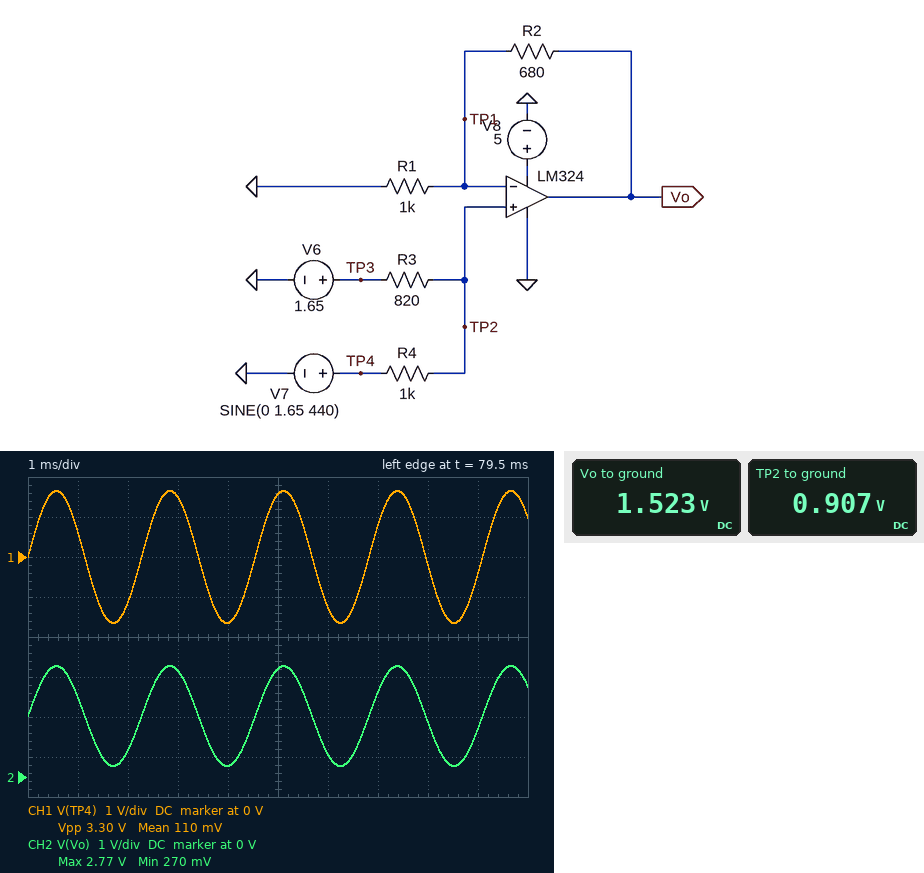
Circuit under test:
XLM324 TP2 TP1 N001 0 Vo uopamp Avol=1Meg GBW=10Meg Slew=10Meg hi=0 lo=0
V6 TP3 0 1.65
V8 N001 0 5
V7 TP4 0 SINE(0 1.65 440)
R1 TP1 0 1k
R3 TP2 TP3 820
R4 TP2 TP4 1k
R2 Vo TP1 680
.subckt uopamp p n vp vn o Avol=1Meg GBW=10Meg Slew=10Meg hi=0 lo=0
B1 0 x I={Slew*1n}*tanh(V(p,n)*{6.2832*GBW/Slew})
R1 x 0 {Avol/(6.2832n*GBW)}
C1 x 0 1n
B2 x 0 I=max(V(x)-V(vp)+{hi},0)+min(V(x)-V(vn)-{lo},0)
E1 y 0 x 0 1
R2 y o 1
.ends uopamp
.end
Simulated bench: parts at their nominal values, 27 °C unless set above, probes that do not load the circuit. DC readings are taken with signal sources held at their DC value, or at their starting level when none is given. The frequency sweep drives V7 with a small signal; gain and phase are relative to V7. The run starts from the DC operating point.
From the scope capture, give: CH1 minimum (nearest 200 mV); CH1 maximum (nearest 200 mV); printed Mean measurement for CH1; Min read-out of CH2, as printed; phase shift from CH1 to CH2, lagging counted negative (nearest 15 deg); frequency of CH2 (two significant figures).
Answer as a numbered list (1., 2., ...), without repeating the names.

1. -1.6 V
2. 1.6 V
3. 110 mV
4. 270 mV
5. 0 deg
6. 440 Hz
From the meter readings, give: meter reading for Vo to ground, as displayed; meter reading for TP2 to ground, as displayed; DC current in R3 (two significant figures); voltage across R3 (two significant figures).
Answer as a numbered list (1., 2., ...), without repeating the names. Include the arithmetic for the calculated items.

1. 1.523 V
2. 0.907 V
3. (1.65 V - 907 mV) / 820 Ω = 910 µA
4. 1.65 V - 907 mV = 740 mV
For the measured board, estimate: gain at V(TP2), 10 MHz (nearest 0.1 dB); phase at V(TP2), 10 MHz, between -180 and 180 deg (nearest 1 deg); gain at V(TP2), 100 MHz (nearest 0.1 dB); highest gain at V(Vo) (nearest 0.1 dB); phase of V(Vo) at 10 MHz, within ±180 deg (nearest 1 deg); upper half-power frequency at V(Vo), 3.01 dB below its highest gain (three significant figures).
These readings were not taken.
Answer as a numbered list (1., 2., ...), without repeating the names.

1. -6.9 dB
2. 0 deg
3. -6.9 dB
4. -2.4 dB
5. -59 deg
6. 5.95 MHz
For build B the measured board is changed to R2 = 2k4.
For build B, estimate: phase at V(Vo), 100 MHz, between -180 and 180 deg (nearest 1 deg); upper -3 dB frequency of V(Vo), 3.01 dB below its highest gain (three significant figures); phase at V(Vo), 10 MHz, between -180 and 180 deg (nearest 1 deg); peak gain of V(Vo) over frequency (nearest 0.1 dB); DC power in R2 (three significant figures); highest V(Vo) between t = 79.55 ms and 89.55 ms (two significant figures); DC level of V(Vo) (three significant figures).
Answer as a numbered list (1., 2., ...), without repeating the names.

1. -88 deg
2. 2.94 MHz
3. -74 deg
4. 3.7 dB
5. 1.97 mW
6. 5.0 V
7. 3.08 V
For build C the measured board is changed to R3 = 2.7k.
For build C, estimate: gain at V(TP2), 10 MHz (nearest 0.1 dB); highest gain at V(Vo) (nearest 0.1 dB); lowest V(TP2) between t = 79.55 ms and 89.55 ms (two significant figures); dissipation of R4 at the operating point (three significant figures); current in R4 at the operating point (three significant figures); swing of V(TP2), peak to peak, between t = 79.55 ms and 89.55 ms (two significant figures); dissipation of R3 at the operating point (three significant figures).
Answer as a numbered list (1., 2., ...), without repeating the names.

1. -2.7 dB
2. 1.8 dB
3. -760 mV
4. 199 µW
5. 446 µA
6. 2.4 V
7. 537 µW
